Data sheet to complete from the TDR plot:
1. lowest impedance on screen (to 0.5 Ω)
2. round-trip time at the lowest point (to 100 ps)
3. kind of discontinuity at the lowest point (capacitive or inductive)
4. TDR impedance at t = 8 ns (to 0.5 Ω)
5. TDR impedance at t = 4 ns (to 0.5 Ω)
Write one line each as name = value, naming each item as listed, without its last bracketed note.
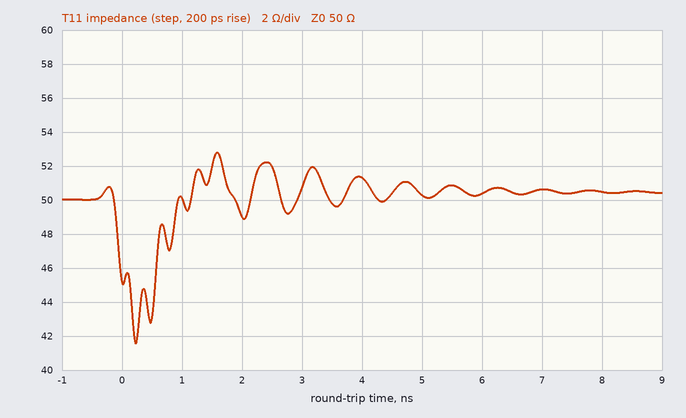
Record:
lowest impedance on screen = 41.5 Ω
round-trip time at the lowest point = 200 ps
kind of discontinuity at the lowest point = capacitive
TDR impedance at t = 8 ns = 50.5 Ω
TDR impedance at t = 4 ns = 51.5 Ω
